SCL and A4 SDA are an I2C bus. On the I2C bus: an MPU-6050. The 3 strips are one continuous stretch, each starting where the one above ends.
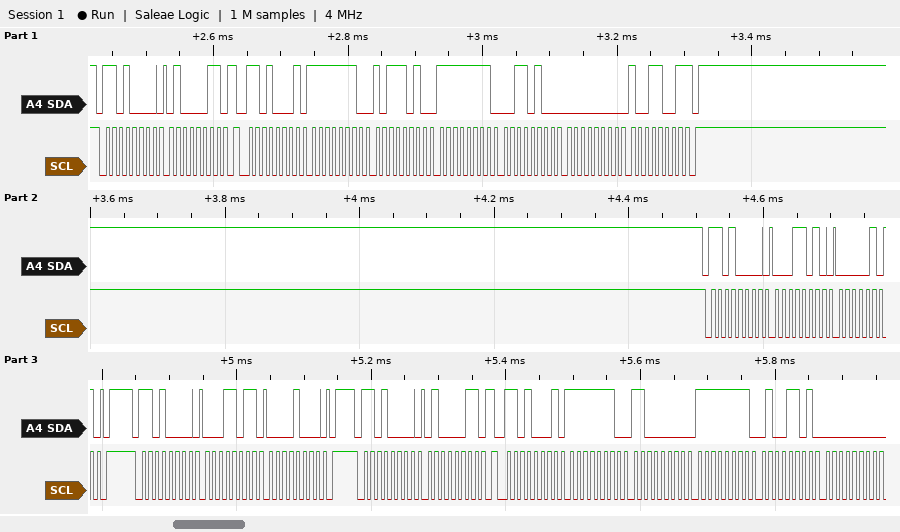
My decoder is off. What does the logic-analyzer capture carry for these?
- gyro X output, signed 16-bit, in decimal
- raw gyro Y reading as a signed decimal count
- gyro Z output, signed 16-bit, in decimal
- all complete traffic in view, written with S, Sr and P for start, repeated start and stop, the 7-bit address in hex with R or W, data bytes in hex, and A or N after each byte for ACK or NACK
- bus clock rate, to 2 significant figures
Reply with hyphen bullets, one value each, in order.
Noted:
- -326
- -204
- 153
- S 68W A 43 A Sr 68R A FE A BA A FF A 34 A 00 A 99 N P S 68W A 1A A 05 A P S 68W A 1B A 08 A P S 68W A 43 A Sr 68R A FE A C0 A FF A 4D A 00 A
- 100 kHz
